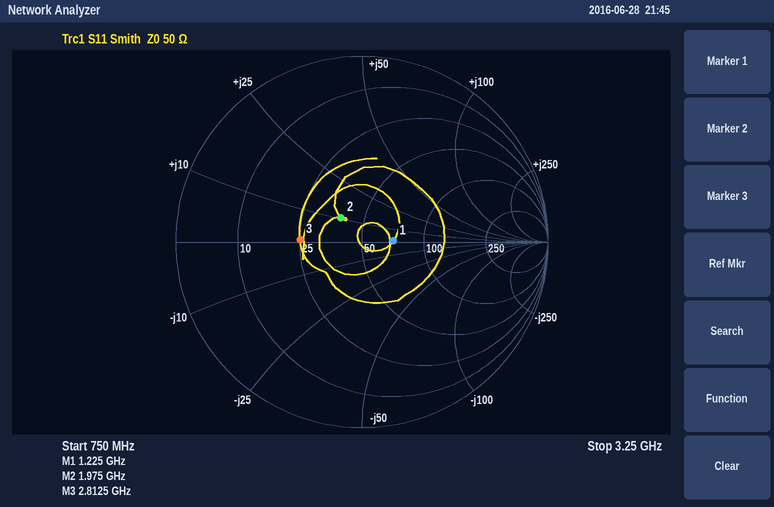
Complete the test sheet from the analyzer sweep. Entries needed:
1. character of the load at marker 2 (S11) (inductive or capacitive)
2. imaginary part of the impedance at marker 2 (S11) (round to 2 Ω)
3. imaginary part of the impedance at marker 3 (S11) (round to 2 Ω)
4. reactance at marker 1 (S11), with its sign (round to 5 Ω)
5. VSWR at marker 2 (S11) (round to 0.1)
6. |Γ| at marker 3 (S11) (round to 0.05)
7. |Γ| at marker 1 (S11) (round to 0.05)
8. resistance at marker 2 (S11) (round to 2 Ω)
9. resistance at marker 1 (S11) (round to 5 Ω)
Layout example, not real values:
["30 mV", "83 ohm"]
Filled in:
["inductive", "+10 Ω", "0 Ω", "0 Ω", "1.4", "0.35", "0.15", "38 Ω", "70 Ω"]
